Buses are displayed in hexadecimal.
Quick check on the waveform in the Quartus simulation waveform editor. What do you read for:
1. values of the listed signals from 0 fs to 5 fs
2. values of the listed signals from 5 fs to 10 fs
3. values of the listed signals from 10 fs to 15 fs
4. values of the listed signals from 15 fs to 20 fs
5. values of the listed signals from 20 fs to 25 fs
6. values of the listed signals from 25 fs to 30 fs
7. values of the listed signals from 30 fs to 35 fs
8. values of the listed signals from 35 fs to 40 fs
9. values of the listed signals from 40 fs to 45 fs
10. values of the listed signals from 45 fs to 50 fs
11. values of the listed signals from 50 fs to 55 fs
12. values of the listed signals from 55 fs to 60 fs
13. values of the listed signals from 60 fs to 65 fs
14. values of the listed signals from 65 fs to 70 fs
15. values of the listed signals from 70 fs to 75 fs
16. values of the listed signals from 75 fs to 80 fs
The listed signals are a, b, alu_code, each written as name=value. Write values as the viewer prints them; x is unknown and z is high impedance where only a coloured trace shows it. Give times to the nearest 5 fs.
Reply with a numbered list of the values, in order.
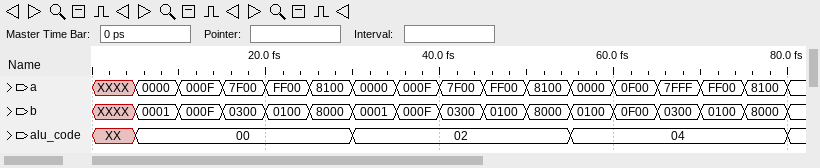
1. a=XXXX, b=XXXX, alu_code=XX
2. a=0000, b=0001, alu_code=00
3. a=000F, b=000F, alu_code=00
4. a=7F00, b=0300, alu_code=00
5. a=FF00, b=0100, alu_code=00
6. a=8100, b=8000, alu_code=00
7. a=0000, b=0001, alu_code=02
8. a=000F, b=000F, alu_code=02
9. a=7F00, b=0300, alu_code=02
10. a=FF00, b=0100, alu_code=02
11. a=8100, b=8000, alu_code=02
12. a=0000, b=0100, alu_code=04
13. a=0F00, b=0F00, alu_code=04
14. a=7FFF, b=0300, alu_code=04
15. a=FF00, b=0100, alu_code=04
16. a=8100, b=8000, alu_code=04
